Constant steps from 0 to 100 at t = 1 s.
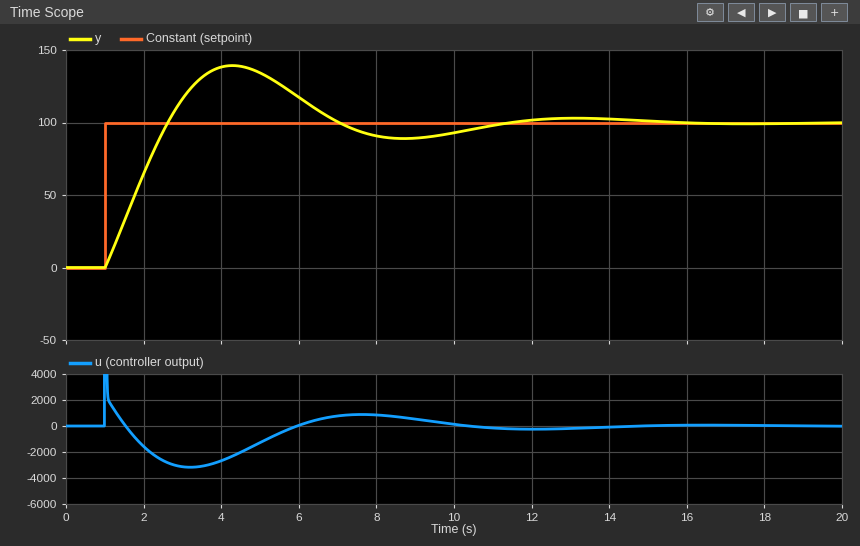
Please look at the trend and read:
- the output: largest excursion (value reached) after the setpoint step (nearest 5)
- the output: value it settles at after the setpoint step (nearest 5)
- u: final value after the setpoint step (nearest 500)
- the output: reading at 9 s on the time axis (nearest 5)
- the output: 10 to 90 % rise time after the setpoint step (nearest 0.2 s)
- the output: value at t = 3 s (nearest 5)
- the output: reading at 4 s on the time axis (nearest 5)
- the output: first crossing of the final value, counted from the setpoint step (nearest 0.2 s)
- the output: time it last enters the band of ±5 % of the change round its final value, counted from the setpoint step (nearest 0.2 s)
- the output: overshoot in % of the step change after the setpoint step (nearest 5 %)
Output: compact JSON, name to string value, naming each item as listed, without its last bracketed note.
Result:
{"the output: largest excursion (value reached) after the setpoint step": "140", "the output: value it settles at after the setpoint step": "100", "u: final value after the setpoint step": "0", "the output: reading at 9 s on the time axis": "90", "the output: 10 to 90 % rise time after the setpoint step": "1.2 s", "the output: value at t = 3 s": "115", "the output: reading at 4 s on the time axis": "140", "the output: first crossing of the final value, counted from the setpoint step": "1.6 s", "the output: time it last enters the band of ±5 % of the change round its final value, counted from the setpoint step": "9.4 s", "the output: overshoot in % of the step change after the setpoint step": "40 %"}
